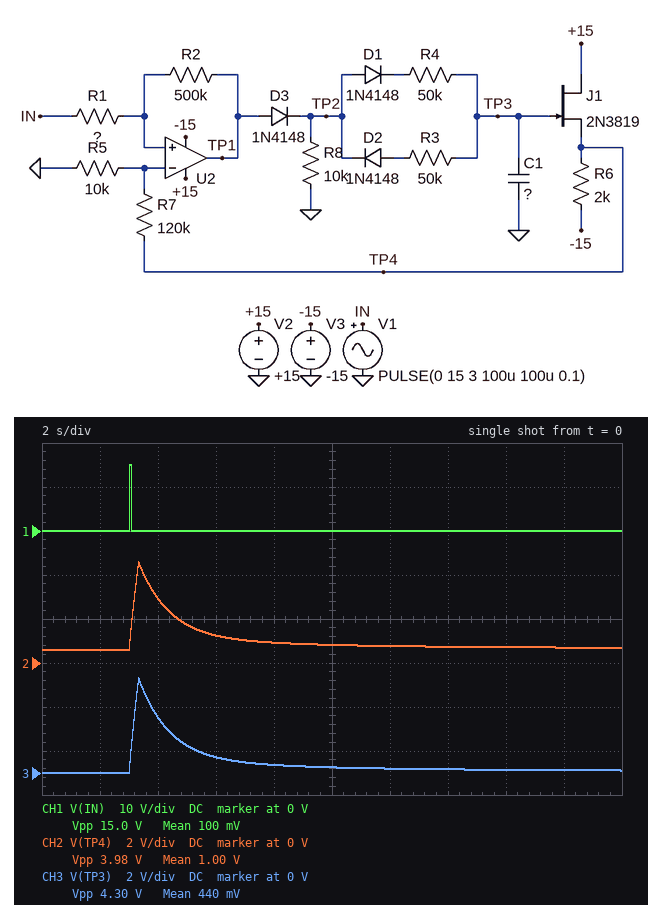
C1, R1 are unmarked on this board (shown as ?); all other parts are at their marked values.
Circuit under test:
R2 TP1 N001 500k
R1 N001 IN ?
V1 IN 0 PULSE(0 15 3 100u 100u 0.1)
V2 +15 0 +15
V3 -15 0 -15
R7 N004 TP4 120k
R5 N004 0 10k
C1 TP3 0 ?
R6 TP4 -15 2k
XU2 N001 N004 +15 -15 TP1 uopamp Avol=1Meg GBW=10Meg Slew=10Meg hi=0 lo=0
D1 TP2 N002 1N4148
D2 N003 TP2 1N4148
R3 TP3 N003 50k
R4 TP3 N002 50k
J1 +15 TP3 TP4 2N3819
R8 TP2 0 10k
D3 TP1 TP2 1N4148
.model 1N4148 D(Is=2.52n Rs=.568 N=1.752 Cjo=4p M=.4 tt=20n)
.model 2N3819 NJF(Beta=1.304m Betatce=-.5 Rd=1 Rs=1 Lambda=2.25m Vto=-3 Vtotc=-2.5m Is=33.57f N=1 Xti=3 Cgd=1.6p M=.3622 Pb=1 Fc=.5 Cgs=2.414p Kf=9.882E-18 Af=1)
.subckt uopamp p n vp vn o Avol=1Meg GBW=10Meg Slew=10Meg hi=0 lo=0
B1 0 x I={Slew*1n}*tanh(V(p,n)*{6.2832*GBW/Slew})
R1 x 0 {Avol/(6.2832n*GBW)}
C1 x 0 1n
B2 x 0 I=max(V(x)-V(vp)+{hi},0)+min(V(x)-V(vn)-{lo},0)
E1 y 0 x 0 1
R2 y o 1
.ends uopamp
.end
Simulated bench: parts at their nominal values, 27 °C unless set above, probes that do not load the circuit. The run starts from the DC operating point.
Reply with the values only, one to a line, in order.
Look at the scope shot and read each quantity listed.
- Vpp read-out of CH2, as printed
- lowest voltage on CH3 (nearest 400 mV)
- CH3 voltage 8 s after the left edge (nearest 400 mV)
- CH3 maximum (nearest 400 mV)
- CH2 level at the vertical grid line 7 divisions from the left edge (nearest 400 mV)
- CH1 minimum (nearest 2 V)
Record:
3.98 V
0 V
400 mV
4.4 V
800 mV
0 V
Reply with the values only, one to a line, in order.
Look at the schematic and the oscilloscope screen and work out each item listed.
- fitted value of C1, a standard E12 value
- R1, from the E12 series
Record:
18 µF
12 kΩ
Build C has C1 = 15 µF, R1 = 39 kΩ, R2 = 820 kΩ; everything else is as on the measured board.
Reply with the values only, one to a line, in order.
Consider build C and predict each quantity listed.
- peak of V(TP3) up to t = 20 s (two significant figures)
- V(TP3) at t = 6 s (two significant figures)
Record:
8.9 V
1.1 V
